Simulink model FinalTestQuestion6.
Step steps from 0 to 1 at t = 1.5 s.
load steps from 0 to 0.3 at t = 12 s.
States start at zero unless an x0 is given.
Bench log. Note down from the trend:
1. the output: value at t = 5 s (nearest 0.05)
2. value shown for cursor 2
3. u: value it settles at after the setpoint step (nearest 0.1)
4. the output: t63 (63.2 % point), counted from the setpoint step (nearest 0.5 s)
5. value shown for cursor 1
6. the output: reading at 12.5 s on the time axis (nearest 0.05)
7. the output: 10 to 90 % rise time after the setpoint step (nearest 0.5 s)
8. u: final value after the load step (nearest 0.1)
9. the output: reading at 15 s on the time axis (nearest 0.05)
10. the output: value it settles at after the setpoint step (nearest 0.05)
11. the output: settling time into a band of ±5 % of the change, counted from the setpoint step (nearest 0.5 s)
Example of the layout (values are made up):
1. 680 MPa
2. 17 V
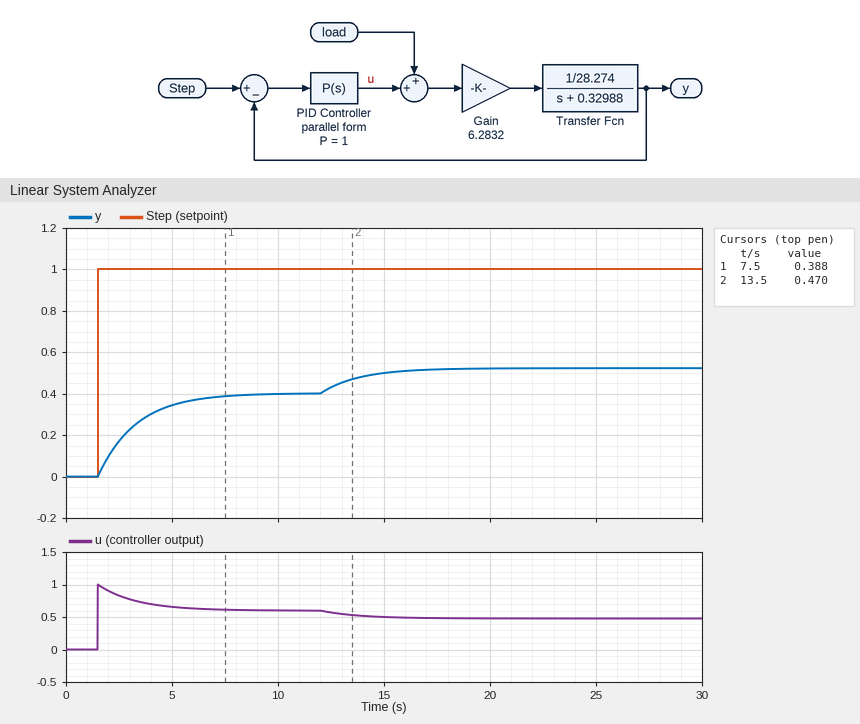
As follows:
1. 0.35
2. 0.470
3. 0.6
4. 2.0 s
5. 0.388
6. 0.45
7. 4.0 s
8. 0.5
9. 0.50
10. 0.40
11. 5.5 s
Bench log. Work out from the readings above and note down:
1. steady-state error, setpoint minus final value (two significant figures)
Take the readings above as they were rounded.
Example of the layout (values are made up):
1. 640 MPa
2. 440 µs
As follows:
1. 0.60
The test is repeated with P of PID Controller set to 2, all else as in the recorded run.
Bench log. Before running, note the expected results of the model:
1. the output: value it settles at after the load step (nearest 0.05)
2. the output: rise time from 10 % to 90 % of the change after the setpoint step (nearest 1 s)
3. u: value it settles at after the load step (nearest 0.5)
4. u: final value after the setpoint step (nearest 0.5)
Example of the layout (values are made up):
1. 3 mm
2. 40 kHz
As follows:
1. 0.65
2. 3 s
3. 0.5
4. 1.0
